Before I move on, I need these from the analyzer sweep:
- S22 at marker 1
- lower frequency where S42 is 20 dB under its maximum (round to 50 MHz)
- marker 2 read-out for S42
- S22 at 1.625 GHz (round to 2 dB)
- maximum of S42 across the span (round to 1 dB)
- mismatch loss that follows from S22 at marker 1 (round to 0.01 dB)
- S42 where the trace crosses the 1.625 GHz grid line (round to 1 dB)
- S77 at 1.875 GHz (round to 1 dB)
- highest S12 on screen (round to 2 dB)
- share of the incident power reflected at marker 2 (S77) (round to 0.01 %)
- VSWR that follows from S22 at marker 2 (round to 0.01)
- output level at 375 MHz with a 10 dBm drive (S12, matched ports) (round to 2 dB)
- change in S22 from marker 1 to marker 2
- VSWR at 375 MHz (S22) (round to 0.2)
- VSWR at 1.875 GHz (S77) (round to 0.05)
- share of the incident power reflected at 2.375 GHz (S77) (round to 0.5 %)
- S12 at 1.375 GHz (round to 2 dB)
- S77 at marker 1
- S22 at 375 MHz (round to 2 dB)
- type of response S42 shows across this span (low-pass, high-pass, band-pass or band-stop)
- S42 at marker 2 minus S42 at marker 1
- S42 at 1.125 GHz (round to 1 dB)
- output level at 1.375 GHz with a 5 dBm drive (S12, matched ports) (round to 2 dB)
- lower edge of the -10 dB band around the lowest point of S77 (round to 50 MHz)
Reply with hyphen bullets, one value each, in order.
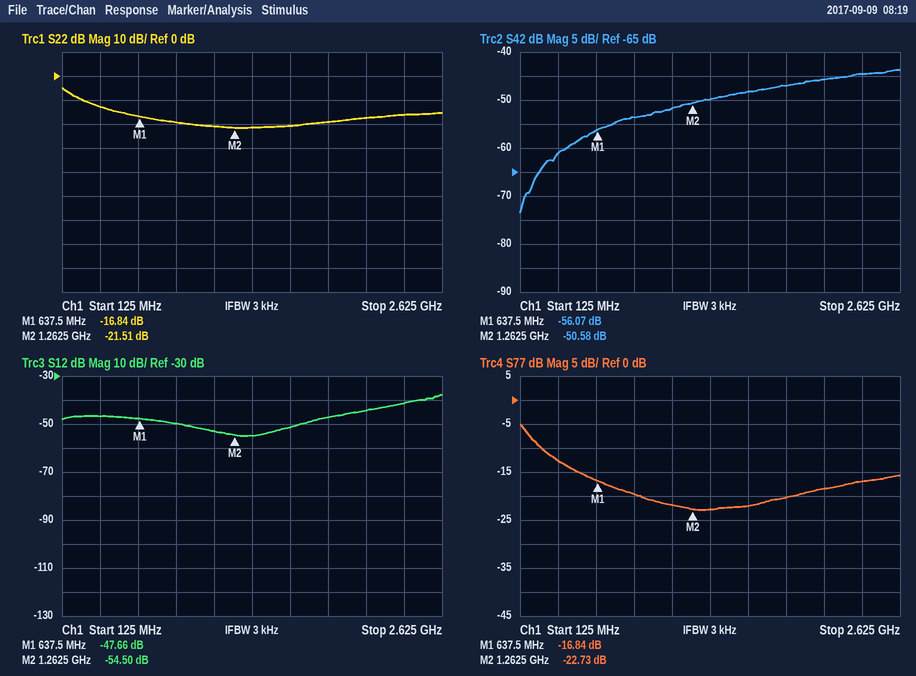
- -16.84 dB
- 300 MHz
- -50.58 dB
- -20 dB
- -44 dB
- 0.09 dB
- -48 dB
- -20 dB
- -38 dB
- 0.53 %
- 1.18
- -36 dBm
- -4.67 dB
- 1.6
- 1.20
- 2.0 %
- -54 dB
- -16.84 dB
- -12 dB
- high-pass
- 5.49 dB
- -52 dB
- -50 dBm
- 250 MHz
